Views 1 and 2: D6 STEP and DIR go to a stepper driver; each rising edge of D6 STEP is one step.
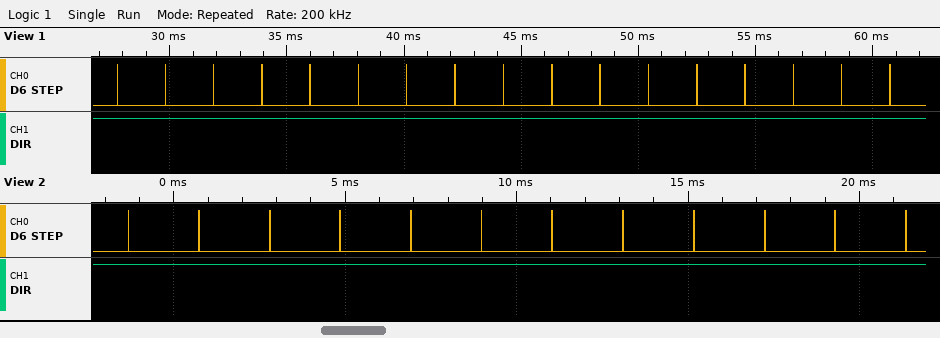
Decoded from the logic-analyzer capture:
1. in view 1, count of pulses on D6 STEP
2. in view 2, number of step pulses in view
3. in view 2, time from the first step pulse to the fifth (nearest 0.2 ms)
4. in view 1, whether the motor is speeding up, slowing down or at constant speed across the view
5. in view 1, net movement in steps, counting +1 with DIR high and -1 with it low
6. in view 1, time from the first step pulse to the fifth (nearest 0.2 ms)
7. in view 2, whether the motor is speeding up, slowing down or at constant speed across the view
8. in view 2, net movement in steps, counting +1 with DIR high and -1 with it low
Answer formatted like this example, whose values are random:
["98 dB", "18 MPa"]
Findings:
["17", "12", "8.2 ms", "constant speed", "+17", "8.2 ms", "constant speed", "+12"]
